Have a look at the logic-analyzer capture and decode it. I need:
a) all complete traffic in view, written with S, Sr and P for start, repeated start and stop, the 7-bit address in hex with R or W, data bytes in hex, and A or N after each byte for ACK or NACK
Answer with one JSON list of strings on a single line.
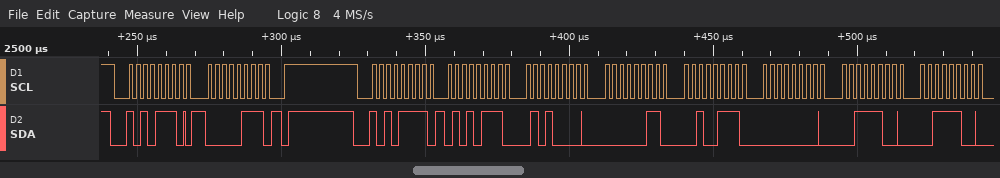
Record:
["S 57W A 07 A P S 57R A 57 A 50 A 03 A 27 A 00 A 3C A 3C A"]
